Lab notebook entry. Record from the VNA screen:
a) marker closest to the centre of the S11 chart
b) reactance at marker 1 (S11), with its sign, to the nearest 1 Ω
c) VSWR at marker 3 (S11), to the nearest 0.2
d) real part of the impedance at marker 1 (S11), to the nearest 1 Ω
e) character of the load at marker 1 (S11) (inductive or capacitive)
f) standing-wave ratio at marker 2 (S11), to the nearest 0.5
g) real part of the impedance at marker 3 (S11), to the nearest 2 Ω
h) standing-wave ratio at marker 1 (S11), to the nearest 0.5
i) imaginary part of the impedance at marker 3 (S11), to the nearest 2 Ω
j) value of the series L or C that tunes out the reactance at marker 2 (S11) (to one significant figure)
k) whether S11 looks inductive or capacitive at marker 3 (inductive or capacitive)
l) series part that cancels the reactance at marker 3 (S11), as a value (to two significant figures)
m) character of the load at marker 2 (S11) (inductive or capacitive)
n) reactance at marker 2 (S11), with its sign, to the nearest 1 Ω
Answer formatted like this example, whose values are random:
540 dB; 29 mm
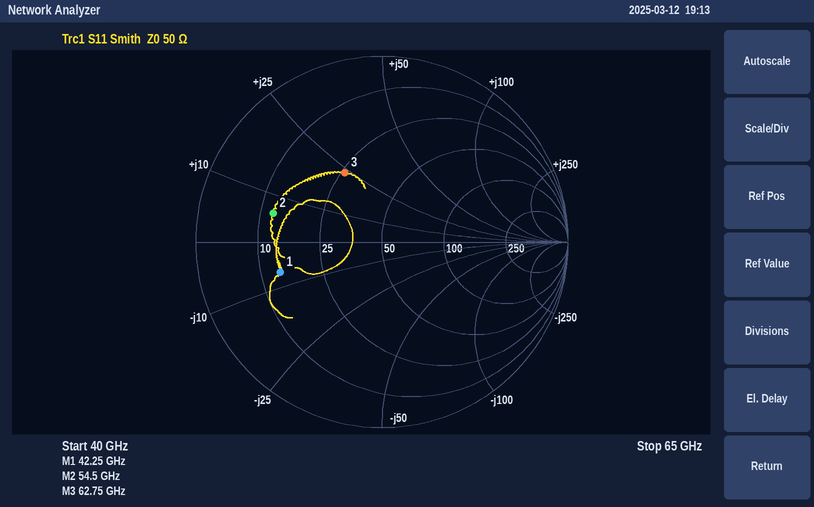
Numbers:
marker 3; -7 Ω; 2.4; 14 Ω; capacitive; 4.0; 26 Ω; 3.5; +24 Ω; 500 fF; inductive; 110 fF; inductive; +6 Ω
